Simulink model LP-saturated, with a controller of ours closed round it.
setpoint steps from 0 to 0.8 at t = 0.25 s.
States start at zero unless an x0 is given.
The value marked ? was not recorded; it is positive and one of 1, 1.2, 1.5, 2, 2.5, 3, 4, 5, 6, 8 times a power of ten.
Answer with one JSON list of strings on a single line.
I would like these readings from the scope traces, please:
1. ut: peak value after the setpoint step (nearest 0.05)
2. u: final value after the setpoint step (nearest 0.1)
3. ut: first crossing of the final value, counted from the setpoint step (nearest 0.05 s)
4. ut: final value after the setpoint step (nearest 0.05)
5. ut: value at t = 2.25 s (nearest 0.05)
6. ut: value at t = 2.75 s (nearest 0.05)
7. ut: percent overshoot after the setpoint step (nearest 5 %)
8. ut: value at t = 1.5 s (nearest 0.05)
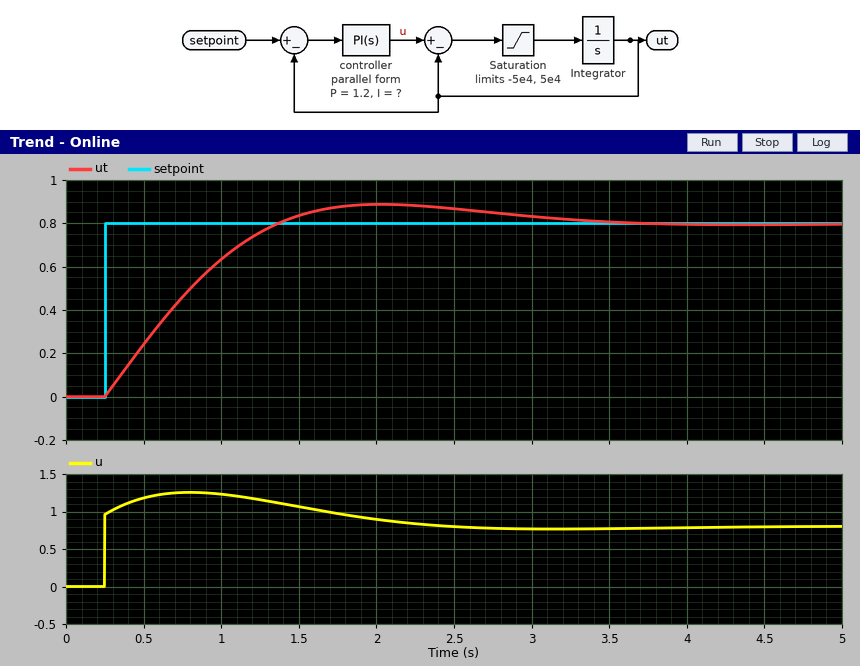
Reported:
["0.90", "0.8", "1.10 s", "0.80", "0.90", "0.85", "10 %", "0.85"]
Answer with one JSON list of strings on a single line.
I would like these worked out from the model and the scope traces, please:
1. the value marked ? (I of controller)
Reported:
["3"]
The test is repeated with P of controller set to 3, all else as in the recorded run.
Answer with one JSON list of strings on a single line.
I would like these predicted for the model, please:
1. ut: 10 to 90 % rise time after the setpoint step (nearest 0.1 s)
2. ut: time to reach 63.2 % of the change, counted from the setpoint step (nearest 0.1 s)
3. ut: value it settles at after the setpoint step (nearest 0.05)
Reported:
["0.7 s", "0.3 s", "0.80"]
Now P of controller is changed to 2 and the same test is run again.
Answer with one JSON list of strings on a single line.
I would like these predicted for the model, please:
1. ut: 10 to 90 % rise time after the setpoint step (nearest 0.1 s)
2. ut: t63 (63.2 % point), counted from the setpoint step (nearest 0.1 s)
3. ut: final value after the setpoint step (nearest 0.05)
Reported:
["0.8 s", "0.4 s", "0.80"]
